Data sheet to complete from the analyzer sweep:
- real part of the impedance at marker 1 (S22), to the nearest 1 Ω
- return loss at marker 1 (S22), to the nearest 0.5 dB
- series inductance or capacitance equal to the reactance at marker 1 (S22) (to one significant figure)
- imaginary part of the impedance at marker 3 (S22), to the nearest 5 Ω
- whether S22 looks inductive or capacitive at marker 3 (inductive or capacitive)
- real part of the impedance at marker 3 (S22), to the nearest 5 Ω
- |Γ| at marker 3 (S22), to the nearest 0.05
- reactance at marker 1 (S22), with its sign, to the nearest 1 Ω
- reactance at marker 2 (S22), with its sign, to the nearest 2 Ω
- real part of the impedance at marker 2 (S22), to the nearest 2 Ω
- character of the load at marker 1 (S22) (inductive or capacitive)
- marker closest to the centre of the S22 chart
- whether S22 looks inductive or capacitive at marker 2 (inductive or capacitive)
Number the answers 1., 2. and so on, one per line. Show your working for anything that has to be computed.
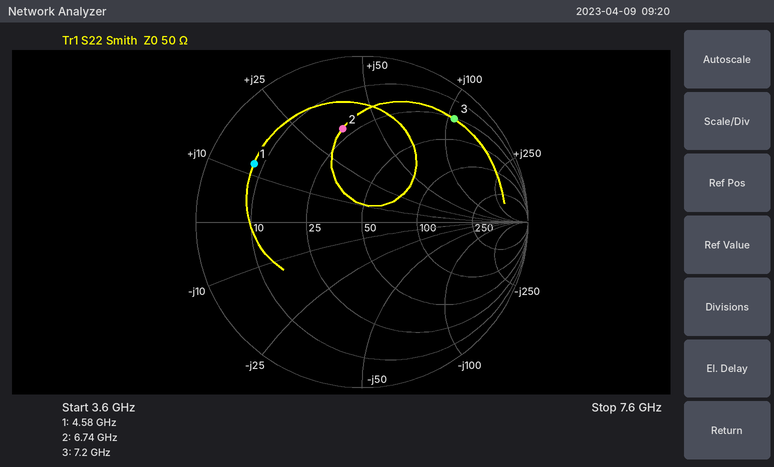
1. 8 Ω
2. 2.5 dB
3. L = 12 Ω/(2π × 4.58 GHz) ≈ 417 pH, so 400 pH to one significant figure
4. +105 Ω
5. inductive
6. 25 Ω
7. 0.85
8. +12 Ω
9. +36 Ω
10. 22 Ω
11. inductive
12. marker 2
13. inductive
